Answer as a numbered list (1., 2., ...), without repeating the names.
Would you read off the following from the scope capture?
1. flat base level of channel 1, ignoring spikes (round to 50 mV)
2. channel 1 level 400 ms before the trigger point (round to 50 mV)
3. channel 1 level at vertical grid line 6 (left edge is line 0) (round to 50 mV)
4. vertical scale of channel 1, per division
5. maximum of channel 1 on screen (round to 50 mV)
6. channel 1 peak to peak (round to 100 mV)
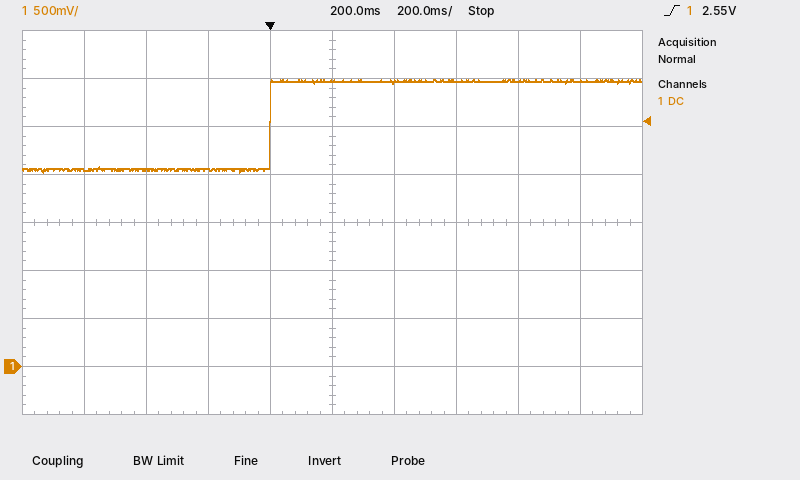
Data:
1. 2.05 V
2. 2.05 V
3. 2.95 V
4. 500 mV
5. 3.00 V
6. 1.00 V
